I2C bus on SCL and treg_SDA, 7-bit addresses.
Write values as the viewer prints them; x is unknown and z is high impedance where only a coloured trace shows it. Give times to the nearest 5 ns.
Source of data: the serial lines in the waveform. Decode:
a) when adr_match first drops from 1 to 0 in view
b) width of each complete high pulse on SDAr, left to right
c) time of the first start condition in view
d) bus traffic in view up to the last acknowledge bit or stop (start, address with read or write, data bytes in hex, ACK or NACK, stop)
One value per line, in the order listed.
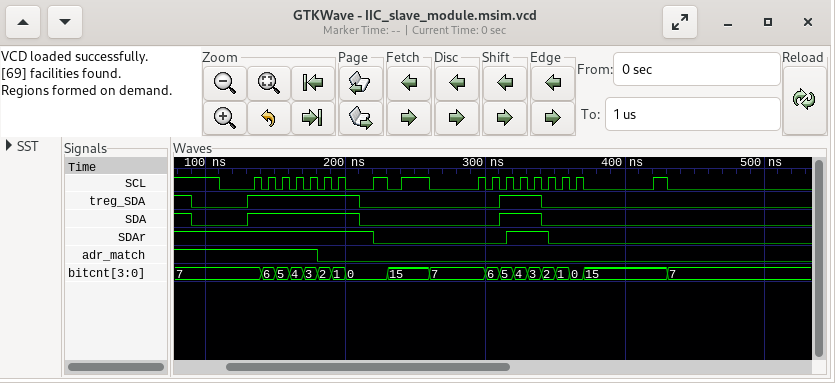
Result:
180 ns
30 ns
90 ns
start, address 7F write ACK, 38 ACK
